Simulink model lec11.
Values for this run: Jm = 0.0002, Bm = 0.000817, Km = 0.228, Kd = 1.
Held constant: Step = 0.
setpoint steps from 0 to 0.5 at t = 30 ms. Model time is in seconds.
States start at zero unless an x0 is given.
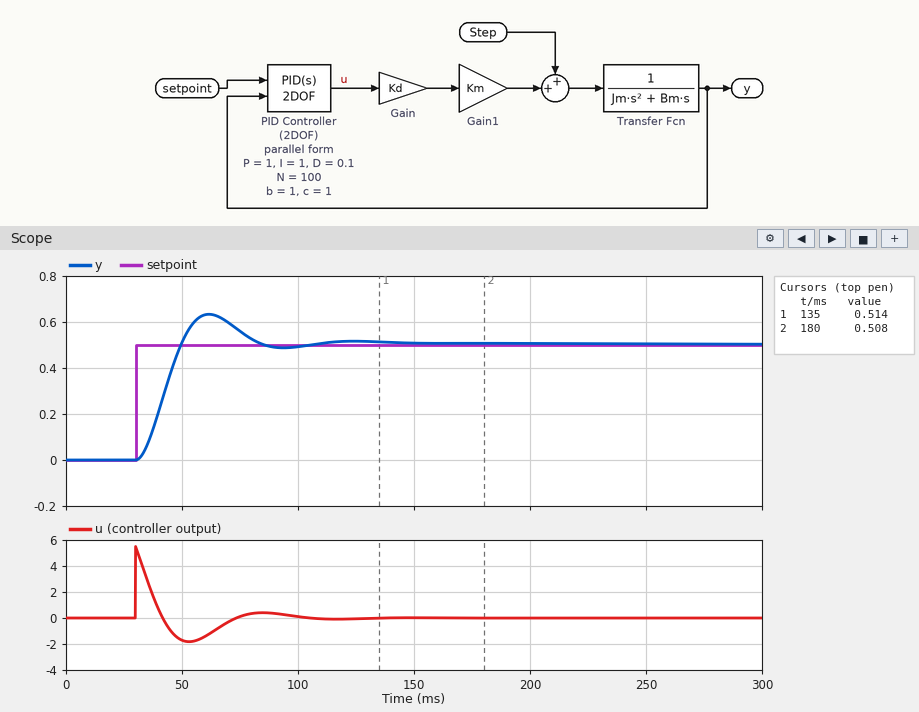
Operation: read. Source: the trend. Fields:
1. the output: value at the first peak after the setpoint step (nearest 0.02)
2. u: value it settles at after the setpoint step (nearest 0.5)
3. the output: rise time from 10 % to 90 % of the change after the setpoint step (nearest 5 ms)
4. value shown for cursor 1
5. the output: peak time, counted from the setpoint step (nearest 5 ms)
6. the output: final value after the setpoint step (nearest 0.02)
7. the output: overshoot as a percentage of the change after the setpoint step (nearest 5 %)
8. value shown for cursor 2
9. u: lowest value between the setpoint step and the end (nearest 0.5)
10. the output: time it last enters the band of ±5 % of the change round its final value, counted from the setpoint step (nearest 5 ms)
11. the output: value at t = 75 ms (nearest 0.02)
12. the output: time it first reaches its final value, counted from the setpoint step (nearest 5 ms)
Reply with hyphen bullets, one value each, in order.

- 0.64
- 0.0
- 15 ms
- 0.514
- 30 ms
- 0.50
- 25 %
- 0.508
- -2.0
- 50 ms
- 0.56
- 20 ms
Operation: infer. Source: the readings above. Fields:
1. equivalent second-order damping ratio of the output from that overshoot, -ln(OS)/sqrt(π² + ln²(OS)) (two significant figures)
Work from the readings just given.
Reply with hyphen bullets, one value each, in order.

- 0.40
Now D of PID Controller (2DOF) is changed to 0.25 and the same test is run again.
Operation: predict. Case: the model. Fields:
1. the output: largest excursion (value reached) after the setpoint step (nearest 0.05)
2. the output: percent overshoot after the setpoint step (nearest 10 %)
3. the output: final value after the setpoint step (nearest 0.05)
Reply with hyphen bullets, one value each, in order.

- 0.70
- 40 %
- 0.50
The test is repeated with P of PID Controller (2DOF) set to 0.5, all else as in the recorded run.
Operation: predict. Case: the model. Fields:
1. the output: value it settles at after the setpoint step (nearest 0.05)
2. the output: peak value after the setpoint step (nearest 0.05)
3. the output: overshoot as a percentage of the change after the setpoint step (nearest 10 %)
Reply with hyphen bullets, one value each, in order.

- 0.50
- 0.60
- 20 %
